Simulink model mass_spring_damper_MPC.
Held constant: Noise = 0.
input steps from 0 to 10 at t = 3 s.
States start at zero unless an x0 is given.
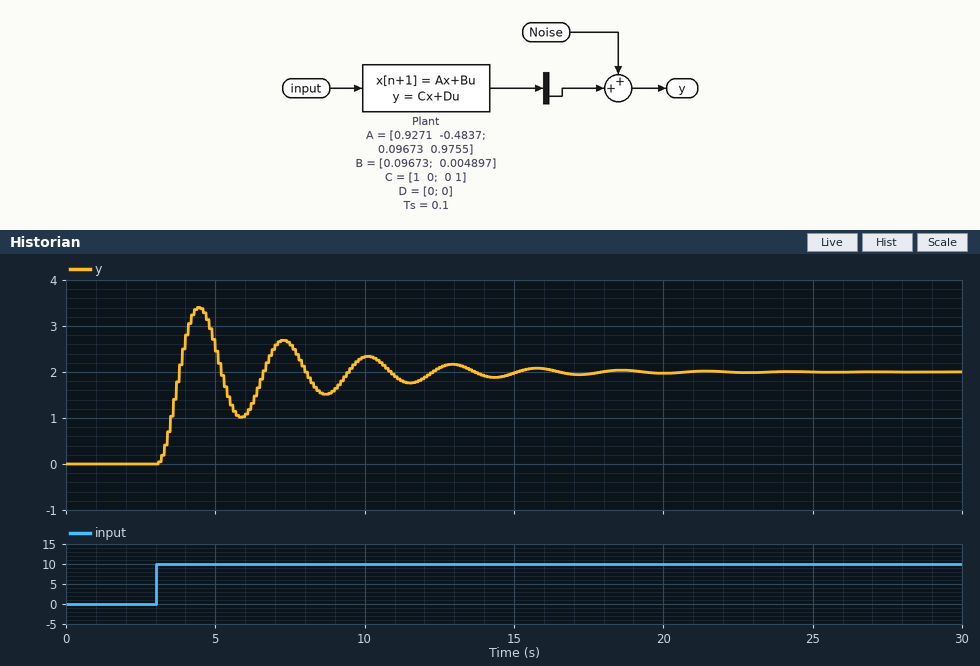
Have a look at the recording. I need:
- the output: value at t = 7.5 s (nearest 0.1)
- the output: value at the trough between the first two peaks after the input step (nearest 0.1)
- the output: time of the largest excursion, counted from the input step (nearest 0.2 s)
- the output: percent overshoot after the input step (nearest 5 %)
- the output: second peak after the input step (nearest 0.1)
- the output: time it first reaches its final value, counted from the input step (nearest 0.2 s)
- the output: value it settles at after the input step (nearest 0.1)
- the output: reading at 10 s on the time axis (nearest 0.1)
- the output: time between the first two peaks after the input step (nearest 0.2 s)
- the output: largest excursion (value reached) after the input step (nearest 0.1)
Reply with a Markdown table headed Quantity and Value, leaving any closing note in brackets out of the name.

| Quantity | Value |
|---|---|
| the output: value at t = 7.5 s | 2.6 |
| the output: value at the trough between the first two peaks after the input step | 1.0 |
| the output: time of the largest excursion, counted from the input step | 1.4 s |
| the output: percent overshoot after the input step | 70 % |
| the output: second peak after the input step | 2.7 |
| the output: time it first reaches its final value, counted from the input step | 0.8 s |
| the output: value it settles at after the input step | 2.0 |
| the output: reading at 10 s on the time axis | 2.3 |
| the output: time between the first two peaks after the input step | 2.8 s |
| the output: largest excursion (value reached) after the input step | 3.4 |
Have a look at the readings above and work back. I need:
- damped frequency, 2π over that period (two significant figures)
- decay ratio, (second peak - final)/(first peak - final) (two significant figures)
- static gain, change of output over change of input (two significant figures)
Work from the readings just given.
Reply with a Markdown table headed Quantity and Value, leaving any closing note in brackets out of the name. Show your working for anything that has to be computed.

| Quantity | Value |
|---|---|
| damped frequency, 2π over that period | 2π / 2.8 = 2.2 rad/s |
| decay ratio, (second peak - final)/(first peak - final) | (2.7 - 2) / (3.4 - 2) = 0.50 |
| static gain, change of output over change of input | (2 - 0) / (10 - 0) = 0.20 |
